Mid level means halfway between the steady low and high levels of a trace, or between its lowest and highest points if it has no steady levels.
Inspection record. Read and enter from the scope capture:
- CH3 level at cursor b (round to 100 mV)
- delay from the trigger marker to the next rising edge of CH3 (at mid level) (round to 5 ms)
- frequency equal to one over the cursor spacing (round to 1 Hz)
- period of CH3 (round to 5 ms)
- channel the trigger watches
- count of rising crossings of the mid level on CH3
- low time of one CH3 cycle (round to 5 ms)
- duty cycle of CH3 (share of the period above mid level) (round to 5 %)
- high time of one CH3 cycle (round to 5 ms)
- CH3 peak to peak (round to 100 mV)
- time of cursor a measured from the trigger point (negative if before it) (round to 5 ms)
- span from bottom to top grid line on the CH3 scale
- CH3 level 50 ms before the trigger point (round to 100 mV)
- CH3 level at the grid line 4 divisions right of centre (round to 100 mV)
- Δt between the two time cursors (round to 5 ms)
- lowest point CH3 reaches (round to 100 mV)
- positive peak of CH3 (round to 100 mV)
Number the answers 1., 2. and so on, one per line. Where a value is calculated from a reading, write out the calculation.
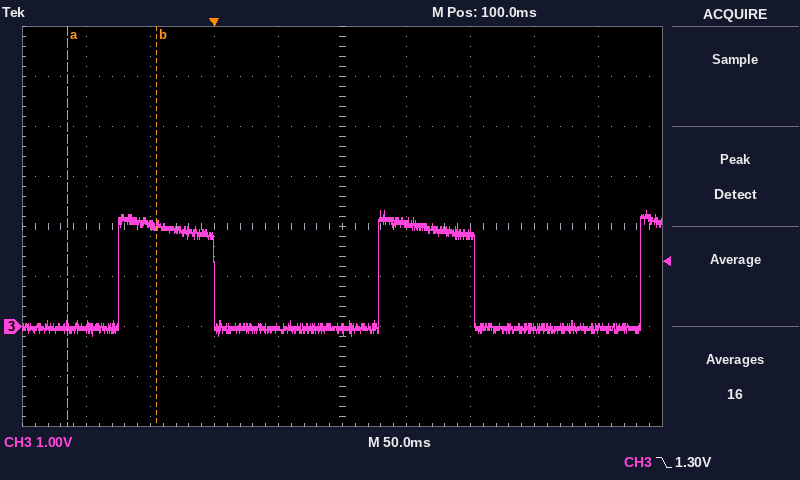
1. 2.0 V
2. 130 ms
3. 1 / 70 ms ≈ 14 Hz
4. 205 ms
5. CH3
6. 3
7. 130 ms
8. 75 ms / 205 ms ≈ 36.6 %, so 35 % to the nearest 5 %
9. 75 ms
10. 2.3 V − (-200 mV) = 2.5 V
11. -115 ms
12. 8 V
13. 2.0 V
14. 0.0 V
15. 70 ms
16. -200 mV
17. 2.3 V
